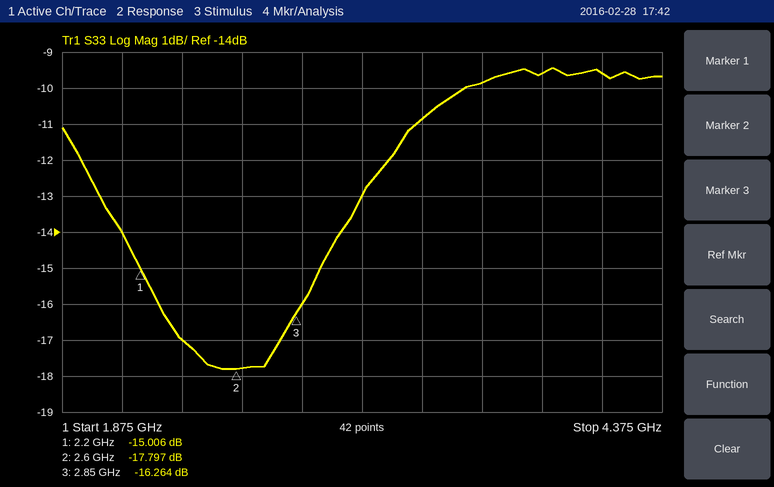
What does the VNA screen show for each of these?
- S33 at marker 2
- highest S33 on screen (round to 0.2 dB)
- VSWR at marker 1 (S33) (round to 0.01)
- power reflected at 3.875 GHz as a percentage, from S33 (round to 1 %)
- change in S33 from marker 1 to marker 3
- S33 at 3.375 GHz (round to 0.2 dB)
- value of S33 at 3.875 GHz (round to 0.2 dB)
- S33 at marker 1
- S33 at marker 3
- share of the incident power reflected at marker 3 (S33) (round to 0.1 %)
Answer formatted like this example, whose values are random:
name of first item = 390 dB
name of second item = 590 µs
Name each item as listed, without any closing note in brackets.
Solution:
S33 at marker 2 = -17.797 dB
highest S33 on screen = -9.4 dB
VSWR at marker 1 (S33) = 1.43
power reflected at 3.875 GHz as a percentage, from S33 = 11 %
change in S33 from marker 1 to marker 3 = -1.258 dB
S33 at 3.375 GHz = -10.8 dB
value of S33 at 3.875 GHz = -9.6 dB
S33 at marker 1 = -15.006 dB
S33 at marker 3 = -16.264 dB
share of the incident power reflected at marker 3 (S33) = 2.4 %
